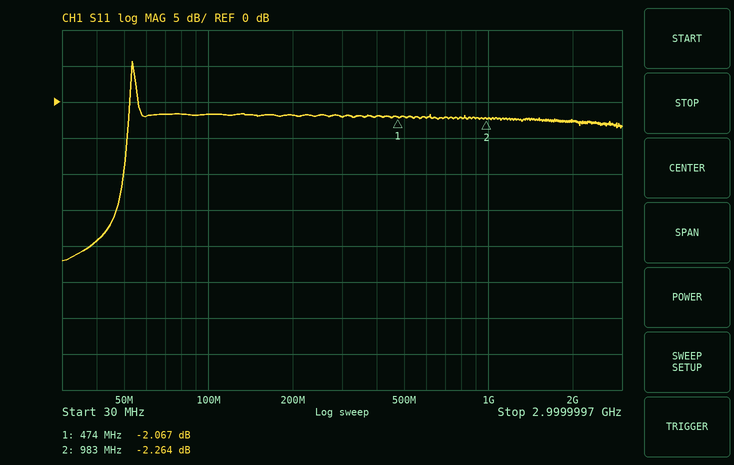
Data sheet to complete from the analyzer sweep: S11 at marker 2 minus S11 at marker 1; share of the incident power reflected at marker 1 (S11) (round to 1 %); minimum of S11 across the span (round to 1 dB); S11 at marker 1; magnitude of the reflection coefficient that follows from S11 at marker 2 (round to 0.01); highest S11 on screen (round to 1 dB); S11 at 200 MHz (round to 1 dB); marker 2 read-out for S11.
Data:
-0.197 dB
62 %
-22 dB
-2.067 dB
0.77
6 dB
-2 dB
-2.264 dB
